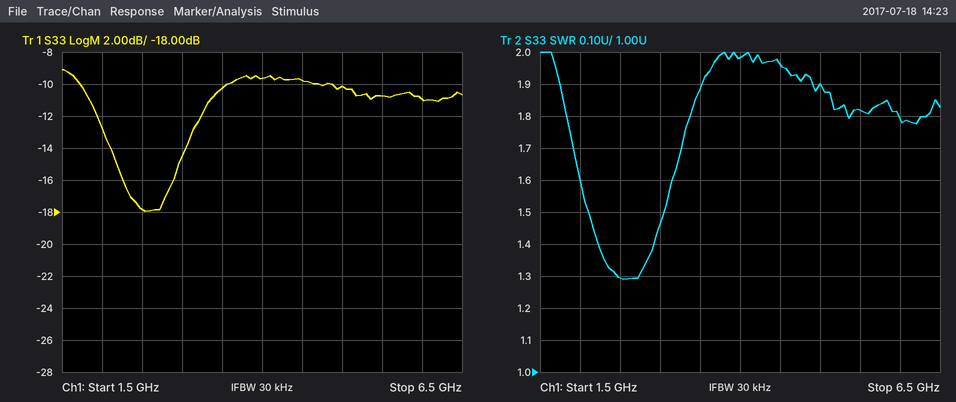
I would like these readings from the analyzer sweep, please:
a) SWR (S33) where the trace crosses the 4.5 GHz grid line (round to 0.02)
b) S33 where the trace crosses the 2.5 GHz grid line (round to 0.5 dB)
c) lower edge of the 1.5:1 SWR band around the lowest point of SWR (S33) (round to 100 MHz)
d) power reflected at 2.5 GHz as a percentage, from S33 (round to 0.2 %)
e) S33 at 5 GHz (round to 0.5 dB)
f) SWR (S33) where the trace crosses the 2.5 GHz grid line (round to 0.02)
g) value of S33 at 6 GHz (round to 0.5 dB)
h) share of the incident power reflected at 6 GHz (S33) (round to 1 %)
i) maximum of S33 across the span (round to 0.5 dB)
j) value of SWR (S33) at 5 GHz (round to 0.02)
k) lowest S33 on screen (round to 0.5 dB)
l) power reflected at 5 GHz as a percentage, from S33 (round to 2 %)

1.96
-18.0 dB
2.1 GHz
1.6 %
-10.0 dB
1.30
-11.0 dB
8 %
-9.0 dB
1.90
-18.0 dB
10 %
